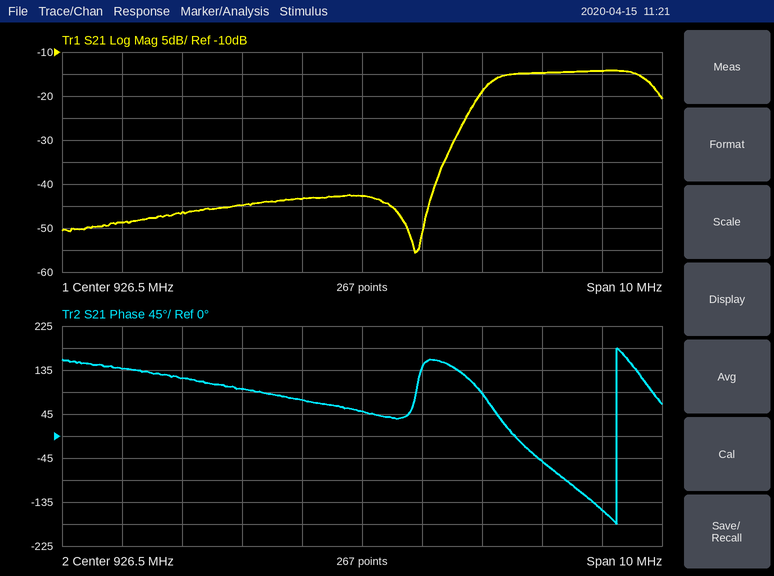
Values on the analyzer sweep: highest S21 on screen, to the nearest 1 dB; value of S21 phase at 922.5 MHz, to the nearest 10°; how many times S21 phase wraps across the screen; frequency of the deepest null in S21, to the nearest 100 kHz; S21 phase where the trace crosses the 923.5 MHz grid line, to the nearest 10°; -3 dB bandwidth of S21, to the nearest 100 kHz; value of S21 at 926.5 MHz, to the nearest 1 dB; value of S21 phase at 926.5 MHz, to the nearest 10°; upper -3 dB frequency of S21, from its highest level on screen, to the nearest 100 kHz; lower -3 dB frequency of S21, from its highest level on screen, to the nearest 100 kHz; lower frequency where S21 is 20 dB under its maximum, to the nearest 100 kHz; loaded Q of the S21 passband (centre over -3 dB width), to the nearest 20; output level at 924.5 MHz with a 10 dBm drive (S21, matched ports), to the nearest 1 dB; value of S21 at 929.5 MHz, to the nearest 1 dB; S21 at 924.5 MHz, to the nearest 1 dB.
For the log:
-14 dB
140°
1
927.4 MHz
120°
2.7 MHz
-43 dB
50°
931.3 MHz
928.6 MHz
927.9 MHz
340
-35 dBm
-15 dB
-45 dB
